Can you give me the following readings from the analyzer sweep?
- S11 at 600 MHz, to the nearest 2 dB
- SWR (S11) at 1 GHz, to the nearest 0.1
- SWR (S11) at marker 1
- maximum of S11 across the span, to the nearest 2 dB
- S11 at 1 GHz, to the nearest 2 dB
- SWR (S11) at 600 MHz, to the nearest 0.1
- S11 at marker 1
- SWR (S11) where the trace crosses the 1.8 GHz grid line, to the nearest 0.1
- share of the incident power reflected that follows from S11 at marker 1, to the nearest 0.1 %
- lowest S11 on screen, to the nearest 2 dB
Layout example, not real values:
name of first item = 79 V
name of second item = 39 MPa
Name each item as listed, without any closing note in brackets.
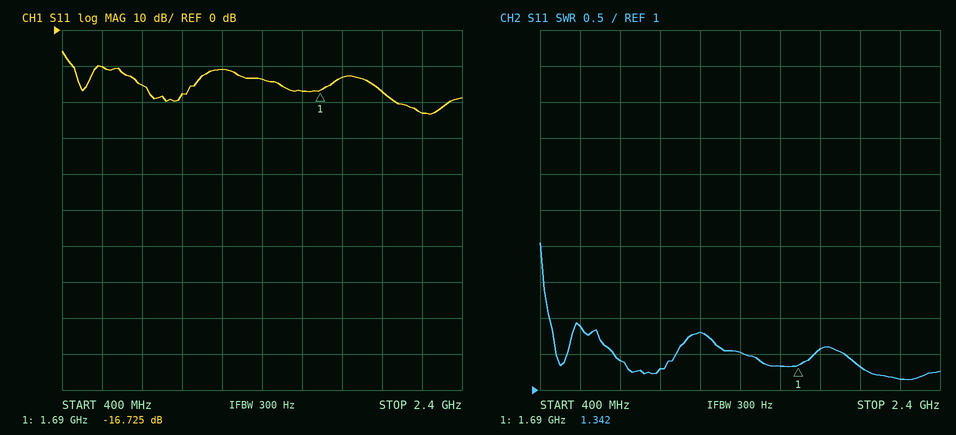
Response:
S11 at 600 MHz, to the nearest 2 dB = -10 dB
SWR (S11) at 1 GHz, to the nearest 0.1 = 1.3
SWR (S11) at marker 1 = 1.342
maximum of S11 across the span, to the nearest 2 dB = -6 dB
S11 at 1 GHz, to the nearest 2 dB = -18 dB
SWR (S11) at 600 MHz, to the nearest 0.1 = 1.9
S11 at marker 1 = -16.725 dB
SWR (S11) where the trace crosses the 1.8 GHz grid line, to the nearest 0.1 = 1.6
share of the incident power reflected that follows from S11 at marker 1, to the nearest 0.1 % = 2.1 %
lowest S11 on screen, to the nearest 2 dB = -24 dB
